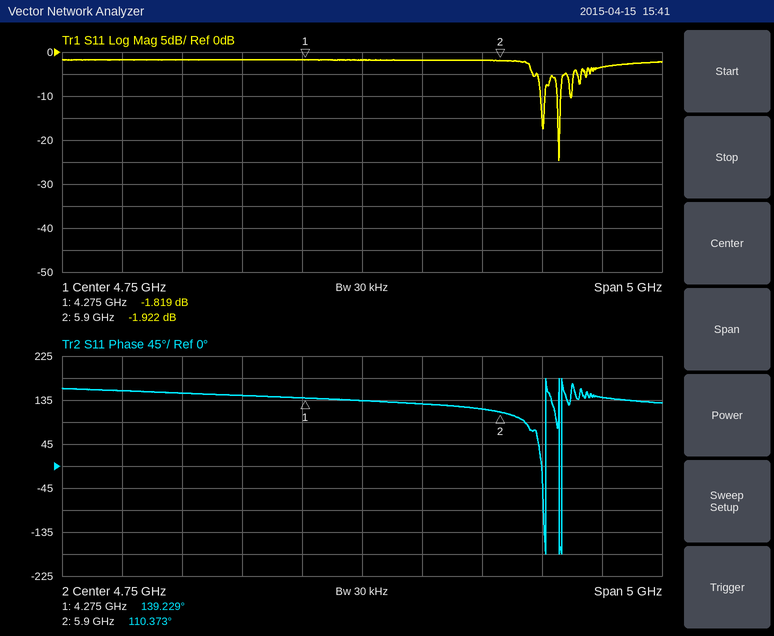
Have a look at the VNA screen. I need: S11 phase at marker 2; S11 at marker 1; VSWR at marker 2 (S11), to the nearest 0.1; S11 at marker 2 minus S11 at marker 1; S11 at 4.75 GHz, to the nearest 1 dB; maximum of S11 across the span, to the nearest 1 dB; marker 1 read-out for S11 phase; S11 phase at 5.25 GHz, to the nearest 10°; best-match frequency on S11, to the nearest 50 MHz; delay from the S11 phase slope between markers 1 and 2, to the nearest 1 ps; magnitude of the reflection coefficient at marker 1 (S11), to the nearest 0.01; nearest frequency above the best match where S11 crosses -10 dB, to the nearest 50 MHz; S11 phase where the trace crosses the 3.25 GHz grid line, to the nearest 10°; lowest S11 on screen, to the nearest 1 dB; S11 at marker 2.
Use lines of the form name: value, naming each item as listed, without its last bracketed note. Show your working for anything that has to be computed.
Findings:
S11 phase at marker 2: 110.373°
S11 at marker 1: -1.819 dB
VSWR at marker 2 (S11), to the nearest 0.1: (1 + 0.8015)/(1 − 0.8015) ≈ 9.1
S11 at marker 2 minus S11 at marker 1: -1.922 − (-1.819) = -0.103 dB
S11 at 4.75 GHz, to the nearest 1 dB: -2 dB
maximum of S11 across the span, to the nearest 1 dB: -2 dB
marker 1 read-out for S11 phase: 139.229°
S11 phase at 5.25 GHz, to the nearest 10°: 130°
best-match frequency on S11, to the nearest 50 MHz: 6.40 GHz
delay from the S11 phase slope between markers 1 and 2, to the nearest 1 ps: −(110.373° − (139.229°))/(360° × 1.625 GHz) ≈ 49 ps
magnitude of the reflection coefficient at marker 1 (S11), to the nearest 0.01: 10^(-1.819/20) ≈ 0.81
nearest frequency above the best match where S11 crosses -10 dB, to the nearest 50 MHz: 6.40 GHz
S11 phase where the trace crosses the 3.25 GHz grid line, to the nearest 10°: 150°
lowest S11 on screen, to the nearest 1 dB: -25 dB
S11 at marker 2: -1.922 dB
